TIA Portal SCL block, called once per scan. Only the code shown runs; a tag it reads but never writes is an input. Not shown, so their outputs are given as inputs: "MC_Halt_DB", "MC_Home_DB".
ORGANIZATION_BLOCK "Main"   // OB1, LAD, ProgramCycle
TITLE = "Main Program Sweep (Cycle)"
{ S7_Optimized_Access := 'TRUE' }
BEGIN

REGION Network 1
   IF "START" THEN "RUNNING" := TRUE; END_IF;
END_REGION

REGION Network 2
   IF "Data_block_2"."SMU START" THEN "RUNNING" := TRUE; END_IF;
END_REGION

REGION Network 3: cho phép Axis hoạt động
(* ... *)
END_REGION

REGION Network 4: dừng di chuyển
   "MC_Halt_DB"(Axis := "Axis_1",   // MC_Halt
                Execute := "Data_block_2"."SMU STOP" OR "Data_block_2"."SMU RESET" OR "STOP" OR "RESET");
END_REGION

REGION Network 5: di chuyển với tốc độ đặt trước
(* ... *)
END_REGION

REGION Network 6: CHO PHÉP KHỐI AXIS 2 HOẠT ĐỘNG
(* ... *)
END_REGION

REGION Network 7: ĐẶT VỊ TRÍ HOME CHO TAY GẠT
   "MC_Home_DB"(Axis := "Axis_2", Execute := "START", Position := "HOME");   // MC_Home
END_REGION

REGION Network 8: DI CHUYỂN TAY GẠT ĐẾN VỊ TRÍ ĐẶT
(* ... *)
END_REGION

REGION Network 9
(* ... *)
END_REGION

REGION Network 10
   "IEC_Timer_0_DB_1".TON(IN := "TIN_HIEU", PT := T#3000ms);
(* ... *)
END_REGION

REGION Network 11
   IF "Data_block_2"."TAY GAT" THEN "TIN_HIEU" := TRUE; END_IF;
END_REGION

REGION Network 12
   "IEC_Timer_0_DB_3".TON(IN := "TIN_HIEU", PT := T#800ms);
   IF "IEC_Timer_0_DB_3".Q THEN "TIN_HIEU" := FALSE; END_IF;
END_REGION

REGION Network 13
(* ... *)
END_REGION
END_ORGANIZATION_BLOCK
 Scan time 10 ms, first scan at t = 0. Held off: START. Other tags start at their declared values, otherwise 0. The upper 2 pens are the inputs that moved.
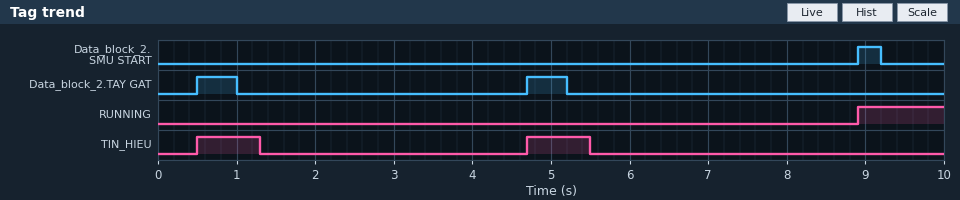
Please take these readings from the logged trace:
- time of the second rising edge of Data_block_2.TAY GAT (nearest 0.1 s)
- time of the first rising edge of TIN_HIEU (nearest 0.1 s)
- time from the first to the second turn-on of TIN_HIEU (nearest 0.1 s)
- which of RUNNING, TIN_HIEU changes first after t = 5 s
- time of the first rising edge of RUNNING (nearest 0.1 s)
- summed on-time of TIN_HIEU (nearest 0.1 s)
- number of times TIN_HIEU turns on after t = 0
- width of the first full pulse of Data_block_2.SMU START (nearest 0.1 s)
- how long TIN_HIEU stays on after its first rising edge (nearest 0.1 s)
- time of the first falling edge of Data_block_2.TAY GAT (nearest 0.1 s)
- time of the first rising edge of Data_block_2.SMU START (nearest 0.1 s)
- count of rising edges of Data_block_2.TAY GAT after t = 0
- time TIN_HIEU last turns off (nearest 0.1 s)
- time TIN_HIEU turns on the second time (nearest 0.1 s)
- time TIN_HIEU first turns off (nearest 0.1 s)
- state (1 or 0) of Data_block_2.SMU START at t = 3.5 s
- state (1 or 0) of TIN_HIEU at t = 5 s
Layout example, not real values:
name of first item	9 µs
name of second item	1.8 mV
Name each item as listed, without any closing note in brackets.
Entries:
time of the second rising edge of Data_block_2.TAY GAT	4.7 s
time of the first rising edge of TIN_HIEU	0.5 s
time from the first to the second turn-on of TIN_HIEU	4.2 s
which of RUNNING, TIN_HIEU changes first after t = 5 s	TIN_HIEU
time of the first rising edge of RUNNING	8.9 s
summed on-time of TIN_HIEU	1.6 s
number of times TIN_HIEU turns on after t = 0	2
width of the first full pulse of Data_block_2.SMU START	0.3 s
how long TIN_HIEU stays on after its first rising edge	0.8 s
time of the first falling edge of Data_block_2.TAY GAT	1.0 s
time of the first rising edge of Data_block_2.SMU START	8.9 s
count of rising edges of Data_block_2.TAY GAT after t = 0	2
time TIN_HIEU last turns off	5.5 s
time TIN_HIEU turns on the second time	4.7 s
time TIN_HIEU first turns off	1.3 s
state (1 or 0) of Data_block_2.SMU START at t = 3.5 s	0
state (1 or 0) of TIN_HIEU at t = 5 s	1
